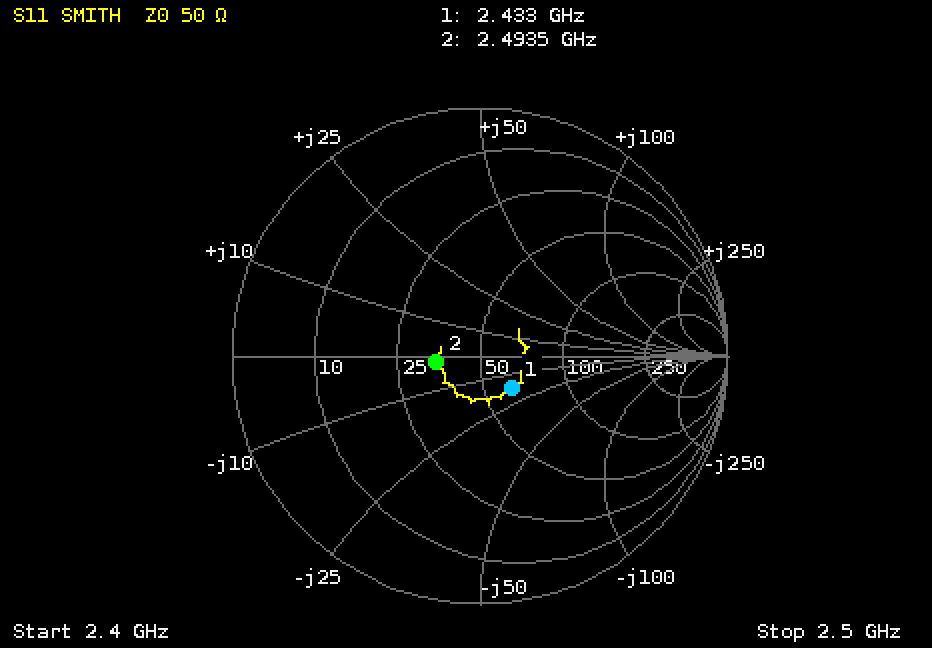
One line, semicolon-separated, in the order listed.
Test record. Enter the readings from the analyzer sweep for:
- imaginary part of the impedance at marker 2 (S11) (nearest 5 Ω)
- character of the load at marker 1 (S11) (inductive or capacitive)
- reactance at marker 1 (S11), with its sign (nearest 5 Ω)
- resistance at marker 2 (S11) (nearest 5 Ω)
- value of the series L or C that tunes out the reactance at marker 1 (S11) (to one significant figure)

0 Ω; capacitive; -15 Ω; 35 Ω; 1 nH
